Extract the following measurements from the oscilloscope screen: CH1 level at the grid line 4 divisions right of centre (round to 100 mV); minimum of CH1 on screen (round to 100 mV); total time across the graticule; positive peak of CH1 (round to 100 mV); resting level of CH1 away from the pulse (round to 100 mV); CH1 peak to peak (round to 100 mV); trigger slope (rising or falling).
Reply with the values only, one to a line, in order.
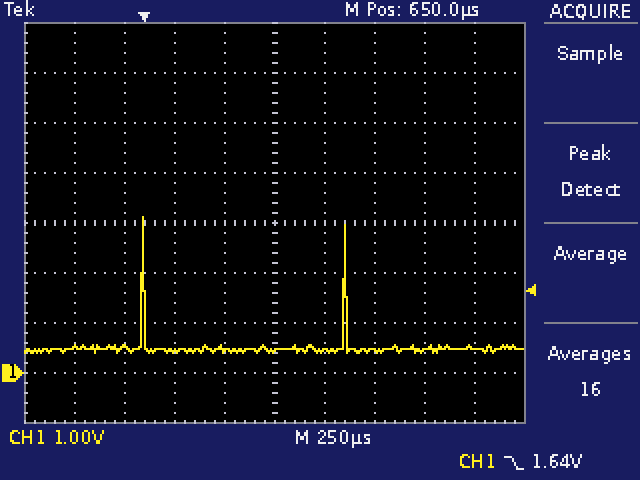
500 mV
400 mV
2.5 ms
3.1 V
500 mV
2.7 V
falling
